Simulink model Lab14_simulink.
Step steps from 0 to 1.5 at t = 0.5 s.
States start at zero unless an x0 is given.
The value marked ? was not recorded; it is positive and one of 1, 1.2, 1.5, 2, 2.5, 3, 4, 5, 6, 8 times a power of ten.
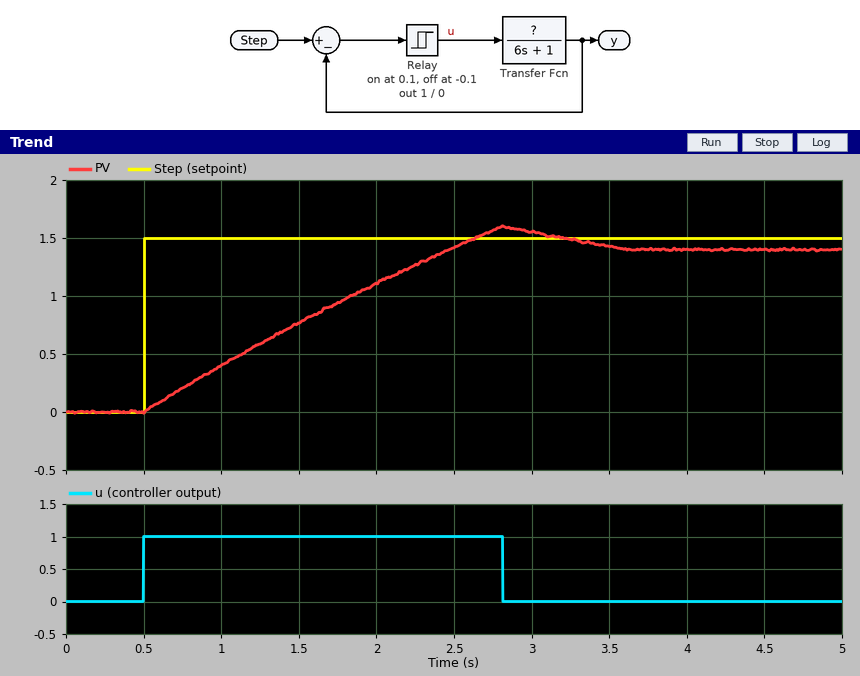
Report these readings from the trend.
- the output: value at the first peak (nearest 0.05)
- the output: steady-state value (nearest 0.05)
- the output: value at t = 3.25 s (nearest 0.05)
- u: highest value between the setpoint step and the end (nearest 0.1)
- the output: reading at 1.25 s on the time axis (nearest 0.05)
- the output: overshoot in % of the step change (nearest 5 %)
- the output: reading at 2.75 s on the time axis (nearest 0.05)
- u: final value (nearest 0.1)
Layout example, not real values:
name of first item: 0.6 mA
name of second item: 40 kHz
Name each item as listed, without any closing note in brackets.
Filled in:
the output: value at the first peak: 1.60
the output: steady-state value: 1.40
the output: value at t = 3.25 s: 1.50
u: highest value between the setpoint step and the end: 1.0
the output: reading at 1.25 s on the time axis: 0.60
the output: overshoot in % of the step change: 15 %
the output: reading at 2.75 s on the time axis: 1.55
u: final value: 0.0
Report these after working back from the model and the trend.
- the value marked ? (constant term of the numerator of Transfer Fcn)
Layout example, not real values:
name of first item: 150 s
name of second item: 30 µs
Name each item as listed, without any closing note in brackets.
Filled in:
the value marked ?: 5
